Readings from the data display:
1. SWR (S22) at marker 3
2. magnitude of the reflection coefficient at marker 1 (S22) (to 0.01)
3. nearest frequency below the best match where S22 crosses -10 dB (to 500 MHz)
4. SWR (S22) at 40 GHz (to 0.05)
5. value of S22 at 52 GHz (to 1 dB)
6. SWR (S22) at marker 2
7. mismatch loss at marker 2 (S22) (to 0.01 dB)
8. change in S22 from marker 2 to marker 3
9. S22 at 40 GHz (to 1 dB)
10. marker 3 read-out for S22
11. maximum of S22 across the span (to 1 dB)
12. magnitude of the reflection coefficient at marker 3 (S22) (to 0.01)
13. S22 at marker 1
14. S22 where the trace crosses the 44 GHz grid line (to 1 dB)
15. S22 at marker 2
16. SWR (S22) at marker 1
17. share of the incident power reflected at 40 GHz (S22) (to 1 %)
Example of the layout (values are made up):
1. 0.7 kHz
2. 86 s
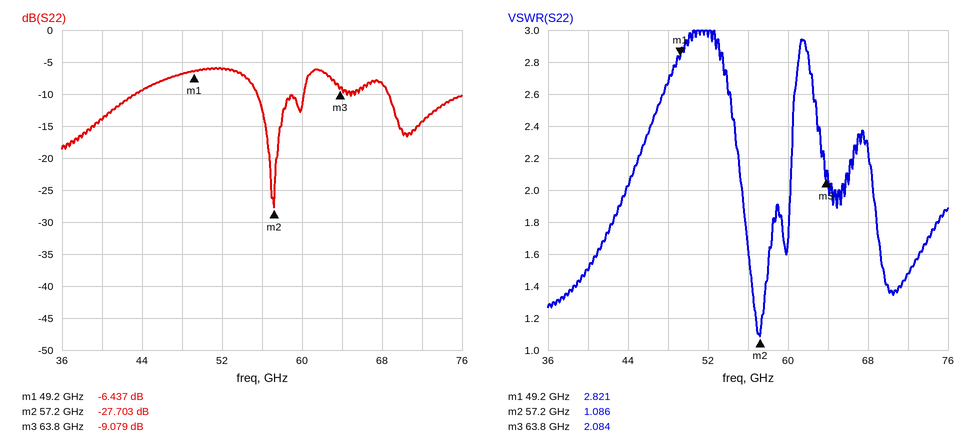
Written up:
1. 2.084
2. 0.48
3. 55.5 GHz
4. 1.50
5. -6 dB
6. 1.086
7. 0.01 dB
8. 18.624 dB
9. -14 dB
10. -9.079 dB
11. -6 dB
12. 0.35
13. -6.437 dB
14. -9 dB
15. -27.703 dB
16. 2.821
17. 4 %
